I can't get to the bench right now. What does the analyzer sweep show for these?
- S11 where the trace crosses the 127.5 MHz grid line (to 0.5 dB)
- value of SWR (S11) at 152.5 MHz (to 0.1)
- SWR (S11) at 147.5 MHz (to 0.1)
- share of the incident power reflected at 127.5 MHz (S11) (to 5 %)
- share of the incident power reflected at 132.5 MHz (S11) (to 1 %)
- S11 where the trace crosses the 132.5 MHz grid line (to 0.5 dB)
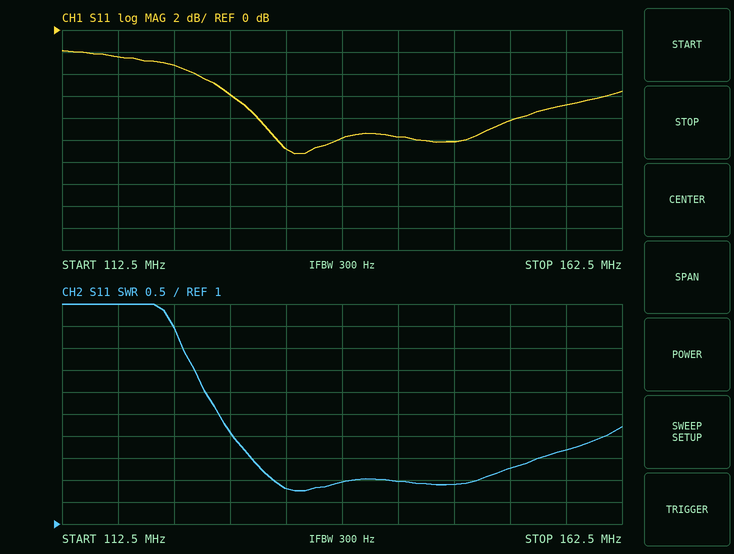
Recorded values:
-6.0 dB
2.3
1.9
25 %
8 %
-11.0 dB
